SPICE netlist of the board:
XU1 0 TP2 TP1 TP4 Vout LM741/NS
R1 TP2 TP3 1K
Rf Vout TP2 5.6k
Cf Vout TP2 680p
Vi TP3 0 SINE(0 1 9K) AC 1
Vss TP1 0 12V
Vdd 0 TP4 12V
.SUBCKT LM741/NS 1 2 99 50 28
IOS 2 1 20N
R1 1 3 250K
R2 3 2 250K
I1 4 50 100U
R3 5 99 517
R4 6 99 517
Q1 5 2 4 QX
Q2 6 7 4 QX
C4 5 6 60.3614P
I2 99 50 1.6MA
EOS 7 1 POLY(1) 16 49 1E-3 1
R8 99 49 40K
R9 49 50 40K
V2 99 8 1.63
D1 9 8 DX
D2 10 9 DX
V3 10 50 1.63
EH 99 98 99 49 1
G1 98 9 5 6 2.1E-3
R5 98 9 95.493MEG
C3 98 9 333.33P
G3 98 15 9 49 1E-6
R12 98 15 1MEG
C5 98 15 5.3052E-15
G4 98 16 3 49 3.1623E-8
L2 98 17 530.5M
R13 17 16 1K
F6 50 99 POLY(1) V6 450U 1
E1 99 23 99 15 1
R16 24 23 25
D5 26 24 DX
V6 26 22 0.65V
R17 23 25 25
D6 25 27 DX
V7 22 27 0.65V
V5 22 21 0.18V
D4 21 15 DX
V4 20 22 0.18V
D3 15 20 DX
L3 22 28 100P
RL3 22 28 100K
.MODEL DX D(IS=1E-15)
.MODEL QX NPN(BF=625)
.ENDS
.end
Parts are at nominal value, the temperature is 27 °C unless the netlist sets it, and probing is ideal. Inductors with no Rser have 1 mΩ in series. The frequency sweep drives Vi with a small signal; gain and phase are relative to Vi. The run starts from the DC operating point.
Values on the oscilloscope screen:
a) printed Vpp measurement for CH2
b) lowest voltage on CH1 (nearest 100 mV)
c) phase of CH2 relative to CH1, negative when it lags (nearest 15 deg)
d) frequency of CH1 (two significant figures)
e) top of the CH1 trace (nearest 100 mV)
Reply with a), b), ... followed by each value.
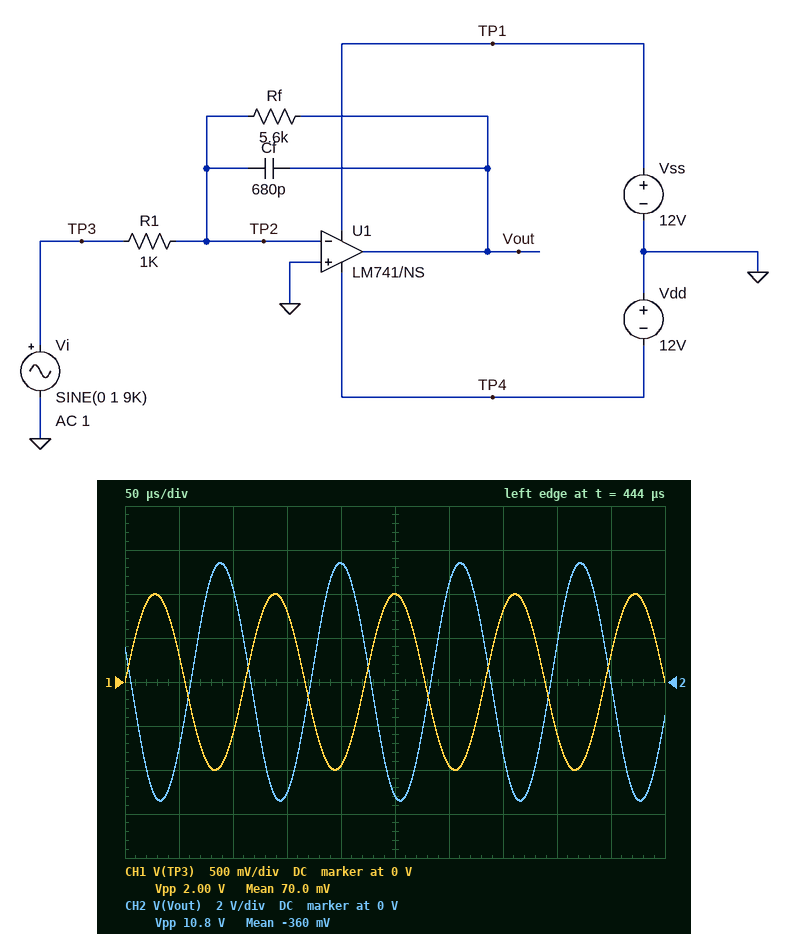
a) 10.8 V
b) -1.0 V
c) 165 deg
d) 9.0 kHz
e) 1.0 V
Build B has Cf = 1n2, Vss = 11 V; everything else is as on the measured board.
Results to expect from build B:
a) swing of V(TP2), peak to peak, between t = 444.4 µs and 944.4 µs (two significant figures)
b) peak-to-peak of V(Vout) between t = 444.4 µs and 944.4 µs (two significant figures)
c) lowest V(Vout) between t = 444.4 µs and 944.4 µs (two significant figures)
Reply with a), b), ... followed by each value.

a) 150 mV
b) 10 V
c) -5.1 V
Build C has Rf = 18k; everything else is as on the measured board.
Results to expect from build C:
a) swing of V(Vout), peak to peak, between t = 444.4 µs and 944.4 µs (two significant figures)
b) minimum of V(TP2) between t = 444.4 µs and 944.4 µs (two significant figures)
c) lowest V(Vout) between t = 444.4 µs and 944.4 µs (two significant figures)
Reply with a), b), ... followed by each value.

a) 16 V
b) -650 mV
c) -8.0 V
